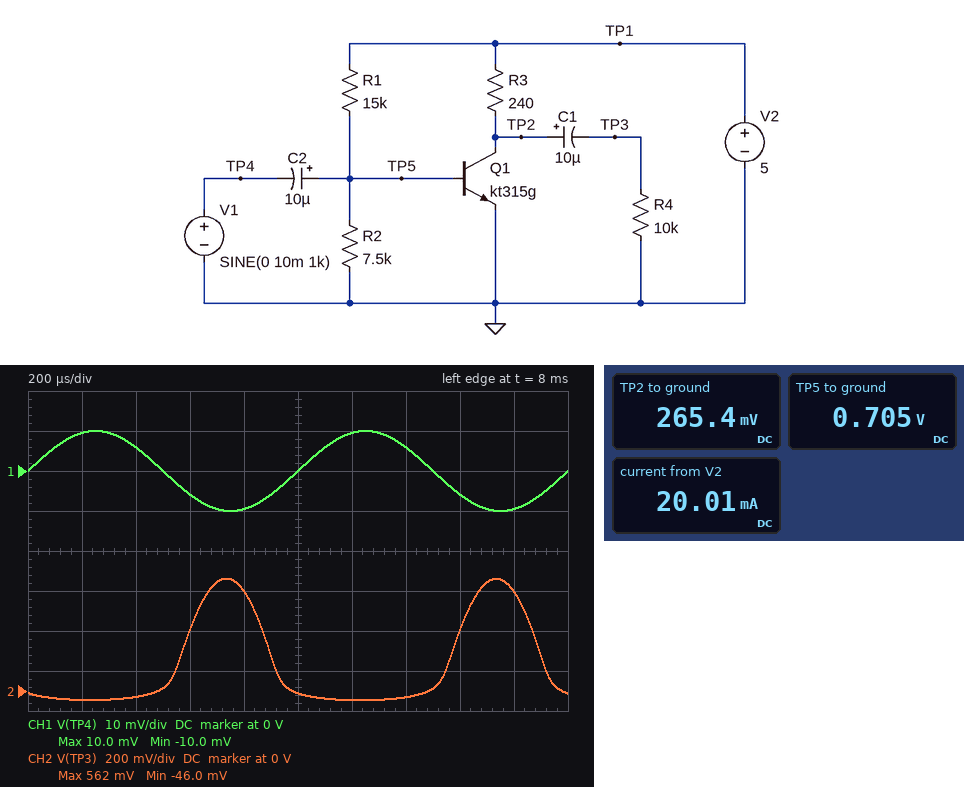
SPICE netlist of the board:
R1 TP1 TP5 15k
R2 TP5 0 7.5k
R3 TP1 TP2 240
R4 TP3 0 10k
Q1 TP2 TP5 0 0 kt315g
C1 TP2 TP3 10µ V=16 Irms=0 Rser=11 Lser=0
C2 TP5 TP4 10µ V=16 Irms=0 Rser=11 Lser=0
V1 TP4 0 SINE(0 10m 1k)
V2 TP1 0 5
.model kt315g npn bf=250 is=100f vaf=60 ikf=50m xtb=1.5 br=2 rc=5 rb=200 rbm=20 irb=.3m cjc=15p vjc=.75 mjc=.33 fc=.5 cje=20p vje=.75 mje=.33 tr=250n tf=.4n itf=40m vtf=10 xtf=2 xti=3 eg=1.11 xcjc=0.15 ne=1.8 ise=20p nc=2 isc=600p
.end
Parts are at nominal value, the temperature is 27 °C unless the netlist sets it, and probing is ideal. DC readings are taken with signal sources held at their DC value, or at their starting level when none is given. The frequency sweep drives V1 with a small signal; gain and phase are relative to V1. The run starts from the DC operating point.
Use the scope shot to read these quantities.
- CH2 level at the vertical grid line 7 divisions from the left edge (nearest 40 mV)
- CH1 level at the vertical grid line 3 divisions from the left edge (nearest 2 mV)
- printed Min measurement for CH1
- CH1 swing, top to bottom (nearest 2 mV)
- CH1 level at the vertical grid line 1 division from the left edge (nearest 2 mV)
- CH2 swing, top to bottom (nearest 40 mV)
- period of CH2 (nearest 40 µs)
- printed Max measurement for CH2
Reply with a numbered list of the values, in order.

1. -40 mV
2. -6 mV
3. -10.0 mV
4. 20 mV
5. 10 mV
6. 600 mV
7. 1.00 ms
8. 562 mV
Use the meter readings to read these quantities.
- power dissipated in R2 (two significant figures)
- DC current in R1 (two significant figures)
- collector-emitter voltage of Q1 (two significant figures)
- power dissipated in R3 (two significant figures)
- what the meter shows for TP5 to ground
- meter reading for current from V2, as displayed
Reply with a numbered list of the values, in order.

1. 66 µW
2. 290 µA
3. 270 mV
4. 93 mW
5. 0.705 V
6. 20.01 mA
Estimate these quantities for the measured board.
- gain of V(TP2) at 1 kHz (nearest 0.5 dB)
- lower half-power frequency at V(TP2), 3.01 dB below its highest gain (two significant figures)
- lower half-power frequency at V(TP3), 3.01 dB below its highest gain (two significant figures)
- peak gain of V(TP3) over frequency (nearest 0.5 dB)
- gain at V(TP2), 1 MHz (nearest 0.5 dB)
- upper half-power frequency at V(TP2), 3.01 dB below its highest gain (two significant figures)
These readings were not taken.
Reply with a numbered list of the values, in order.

1. 15.0 dB
2. 110 Hz
3. 110 Hz
4. 15.0 dB
5. 7.5 dB
6. 440 kHz
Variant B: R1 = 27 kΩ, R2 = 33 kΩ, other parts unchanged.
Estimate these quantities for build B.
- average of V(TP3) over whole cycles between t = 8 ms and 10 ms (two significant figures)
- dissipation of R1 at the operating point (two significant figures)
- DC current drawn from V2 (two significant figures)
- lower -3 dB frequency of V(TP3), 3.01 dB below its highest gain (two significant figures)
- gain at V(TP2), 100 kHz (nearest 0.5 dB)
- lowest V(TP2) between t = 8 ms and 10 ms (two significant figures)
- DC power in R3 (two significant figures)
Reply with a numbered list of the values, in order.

1. 120 mV
2. 690 µW
3. 18 mA
4. 45 Hz
5. 37.0 dB
6. 280 mV
7. 76 mW
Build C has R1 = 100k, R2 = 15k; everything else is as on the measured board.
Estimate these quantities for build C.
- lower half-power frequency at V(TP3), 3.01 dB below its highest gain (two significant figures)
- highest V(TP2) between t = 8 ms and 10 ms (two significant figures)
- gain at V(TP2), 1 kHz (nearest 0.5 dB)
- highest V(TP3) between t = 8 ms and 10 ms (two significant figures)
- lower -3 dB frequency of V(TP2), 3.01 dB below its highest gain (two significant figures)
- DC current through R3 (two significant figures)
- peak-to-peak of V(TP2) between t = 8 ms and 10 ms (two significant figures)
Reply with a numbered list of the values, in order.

1. 4.2 Hz
2. 4.9 V
3. 11.5 dB
4. 32 mV
5. 3.6 Hz
6. 440 µA
7. 77 mV
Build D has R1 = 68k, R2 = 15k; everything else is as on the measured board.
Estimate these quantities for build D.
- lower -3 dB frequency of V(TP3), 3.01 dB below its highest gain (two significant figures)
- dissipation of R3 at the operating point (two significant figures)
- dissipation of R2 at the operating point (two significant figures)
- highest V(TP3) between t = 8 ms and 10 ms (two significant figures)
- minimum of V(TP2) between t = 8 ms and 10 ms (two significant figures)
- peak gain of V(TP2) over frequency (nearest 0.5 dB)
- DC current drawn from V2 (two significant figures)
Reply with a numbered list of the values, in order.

1. 11 Hz
2. 1.7 mW
3. 26 µW
4. 180 mV
5. 4.1 V
6. 26.0 dB
7. 2.7 mA
